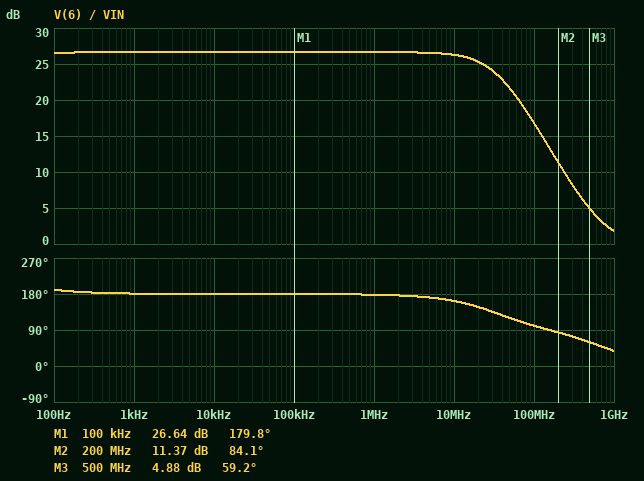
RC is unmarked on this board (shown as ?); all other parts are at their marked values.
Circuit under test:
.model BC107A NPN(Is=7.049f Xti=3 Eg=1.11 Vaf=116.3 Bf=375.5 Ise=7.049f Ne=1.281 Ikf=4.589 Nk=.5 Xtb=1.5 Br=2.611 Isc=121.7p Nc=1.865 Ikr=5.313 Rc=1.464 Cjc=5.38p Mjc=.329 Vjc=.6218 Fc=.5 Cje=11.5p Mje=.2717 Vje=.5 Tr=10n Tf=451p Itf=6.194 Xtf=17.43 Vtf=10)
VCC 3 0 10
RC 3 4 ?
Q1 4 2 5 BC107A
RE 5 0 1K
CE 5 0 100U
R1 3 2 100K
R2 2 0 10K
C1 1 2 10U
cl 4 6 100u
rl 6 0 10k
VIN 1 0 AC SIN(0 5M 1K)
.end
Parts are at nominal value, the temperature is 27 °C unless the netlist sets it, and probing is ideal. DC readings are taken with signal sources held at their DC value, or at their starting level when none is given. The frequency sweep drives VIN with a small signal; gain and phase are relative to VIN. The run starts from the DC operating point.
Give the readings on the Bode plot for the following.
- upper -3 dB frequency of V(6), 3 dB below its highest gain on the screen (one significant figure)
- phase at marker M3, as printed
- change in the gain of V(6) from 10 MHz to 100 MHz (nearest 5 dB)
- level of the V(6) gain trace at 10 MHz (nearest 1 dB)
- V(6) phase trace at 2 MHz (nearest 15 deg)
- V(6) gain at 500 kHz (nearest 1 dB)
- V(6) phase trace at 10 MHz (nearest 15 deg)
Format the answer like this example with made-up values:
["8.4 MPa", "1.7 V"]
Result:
["30 MHz", "59.2 deg", "-10 dB", "26 dB", "180 deg", "27 dB", "165 deg"]
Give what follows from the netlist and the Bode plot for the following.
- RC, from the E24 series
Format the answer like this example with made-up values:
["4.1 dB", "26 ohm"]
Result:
["2.7 kΩ"]
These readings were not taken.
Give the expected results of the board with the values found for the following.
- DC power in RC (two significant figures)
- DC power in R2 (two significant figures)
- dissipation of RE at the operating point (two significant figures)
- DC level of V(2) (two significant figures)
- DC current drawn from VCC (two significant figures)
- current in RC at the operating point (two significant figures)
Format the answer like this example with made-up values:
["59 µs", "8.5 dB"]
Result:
["190 µW", "80 µW", "70 µW", "890 mV", "350 µA", "260 µA"]
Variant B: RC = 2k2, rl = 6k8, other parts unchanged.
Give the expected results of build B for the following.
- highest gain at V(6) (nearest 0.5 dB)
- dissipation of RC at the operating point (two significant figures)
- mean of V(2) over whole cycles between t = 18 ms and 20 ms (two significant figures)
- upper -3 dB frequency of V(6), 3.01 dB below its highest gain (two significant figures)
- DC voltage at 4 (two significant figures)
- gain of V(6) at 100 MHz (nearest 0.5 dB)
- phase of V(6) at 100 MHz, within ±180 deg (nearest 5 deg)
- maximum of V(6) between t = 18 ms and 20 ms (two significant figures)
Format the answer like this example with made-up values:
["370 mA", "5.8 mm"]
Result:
["24.5 dB", "150 µW", "890 mV", "43 MHz", "9.4 V", "16.5 dB", "105 deg", "79 mV"]
